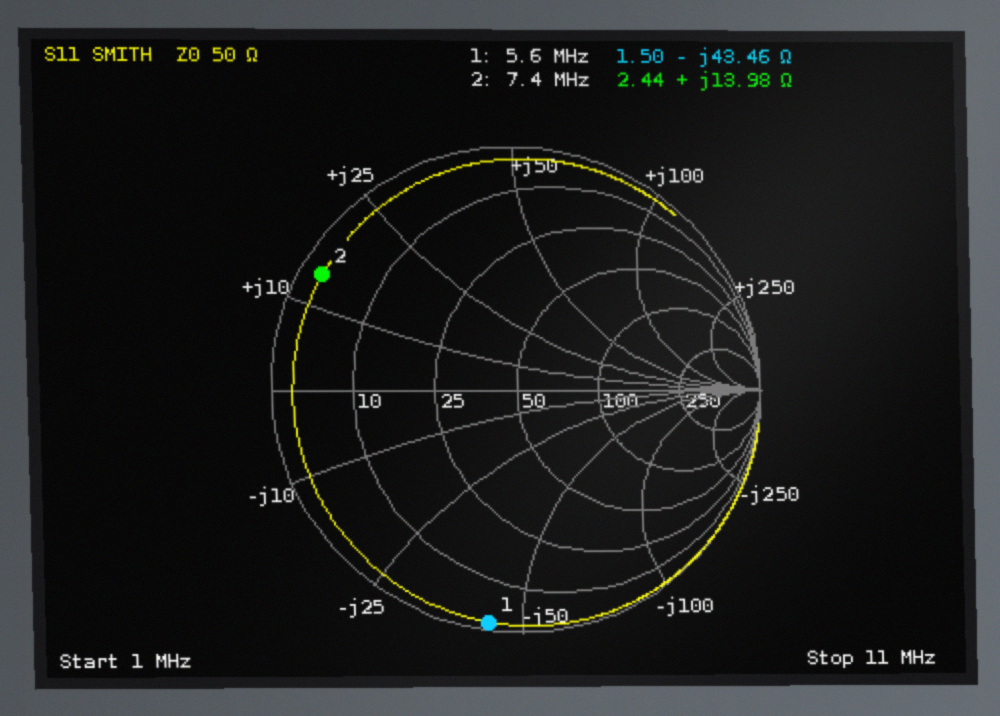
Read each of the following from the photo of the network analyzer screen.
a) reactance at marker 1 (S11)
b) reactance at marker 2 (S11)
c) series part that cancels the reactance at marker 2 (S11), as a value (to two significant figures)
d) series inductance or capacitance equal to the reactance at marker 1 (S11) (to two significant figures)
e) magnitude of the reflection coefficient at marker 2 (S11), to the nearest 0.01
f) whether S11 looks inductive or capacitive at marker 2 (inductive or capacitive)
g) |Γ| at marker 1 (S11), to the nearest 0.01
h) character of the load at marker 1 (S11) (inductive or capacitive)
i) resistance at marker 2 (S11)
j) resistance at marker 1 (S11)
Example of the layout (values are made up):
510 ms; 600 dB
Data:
-43.46 Ω; +13.98 Ω; 1.5 nF; 650 pF; 0.91; inductive; 0.97; capacitive; 2.44 Ω; 1.50 Ω
